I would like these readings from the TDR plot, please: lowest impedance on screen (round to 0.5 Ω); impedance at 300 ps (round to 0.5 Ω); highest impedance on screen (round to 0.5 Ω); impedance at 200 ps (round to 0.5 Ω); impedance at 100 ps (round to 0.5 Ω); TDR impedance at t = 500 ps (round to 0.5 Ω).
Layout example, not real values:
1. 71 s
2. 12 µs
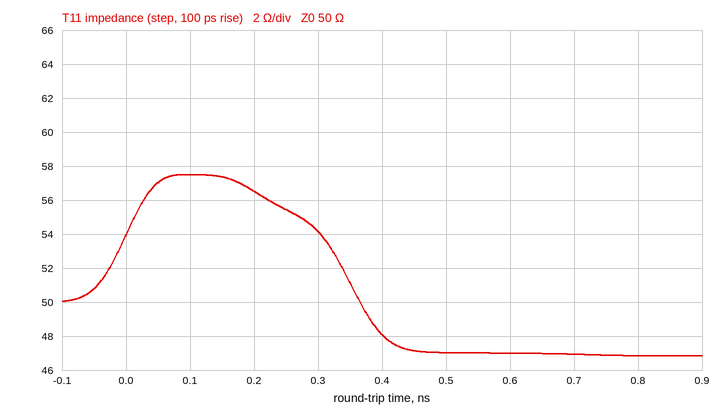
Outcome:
1. 47.0 Ω
2. 54.0 Ω
3. 57.5 Ω
4. 56.5 Ω
5. 57.5 Ω
6. 47.0 Ω
